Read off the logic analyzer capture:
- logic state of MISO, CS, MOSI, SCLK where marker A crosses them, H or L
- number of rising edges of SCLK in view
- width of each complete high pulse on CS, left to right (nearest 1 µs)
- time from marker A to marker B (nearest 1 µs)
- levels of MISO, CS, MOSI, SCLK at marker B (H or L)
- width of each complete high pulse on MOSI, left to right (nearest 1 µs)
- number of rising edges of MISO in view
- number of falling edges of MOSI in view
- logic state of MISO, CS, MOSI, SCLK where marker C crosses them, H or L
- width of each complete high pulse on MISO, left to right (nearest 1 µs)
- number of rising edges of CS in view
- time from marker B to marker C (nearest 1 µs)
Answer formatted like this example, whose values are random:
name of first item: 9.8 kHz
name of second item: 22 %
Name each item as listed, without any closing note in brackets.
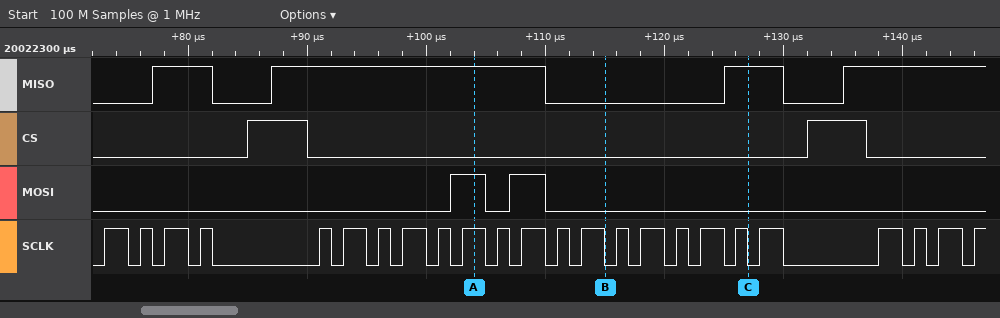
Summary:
logic state of MISO, CS, MOSI, SCLK where marker A crosses them, H or L: MISO=H, CS=L, MOSI=H, SCLK=H
number of rising edges of SCLK in view: 24
width of each complete high pulse on CS, left to right: 5 µs, 5 µs
time from marker A to marker B: 11 µs
levels of MISO, CS, MOSI, SCLK at marker B: MISO=L, CS=L, MOSI=L, SCLK=L
width of each complete high pulse on MOSI, left to right: 3 µs, 3 µs
number of rising edges of MISO in view: 4
number of falling edges of MOSI in view: 2
logic state of MISO, CS, MOSI, SCLK where marker C crosses them, H or L: MISO=H, CS=L, MOSI=L, SCLK=L
width of each complete high pulse on MISO, left to right: 5 µs, 23 µs, 5 µs
number of rising edges of CS in view: 2
time from marker B to marker C: 12 µs
